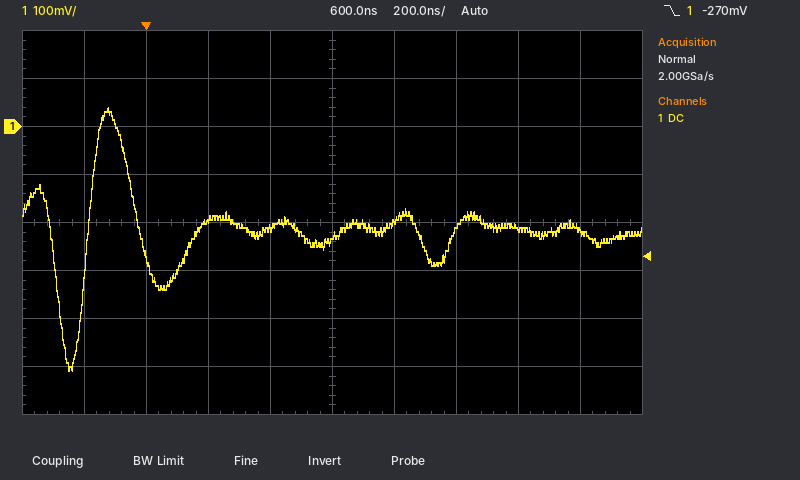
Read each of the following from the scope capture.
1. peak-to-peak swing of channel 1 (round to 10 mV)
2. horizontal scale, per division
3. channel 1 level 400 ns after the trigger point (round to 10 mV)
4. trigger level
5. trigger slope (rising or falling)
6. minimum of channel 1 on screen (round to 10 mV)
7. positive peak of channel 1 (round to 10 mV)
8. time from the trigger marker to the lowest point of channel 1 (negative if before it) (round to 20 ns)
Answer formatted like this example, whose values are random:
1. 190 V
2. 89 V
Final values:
1. 550 mV
2. 200 ns
3. -210 mV
4. -270 mV
5. falling
6. -510 mV
7. 40 mV
8. -240 ns
